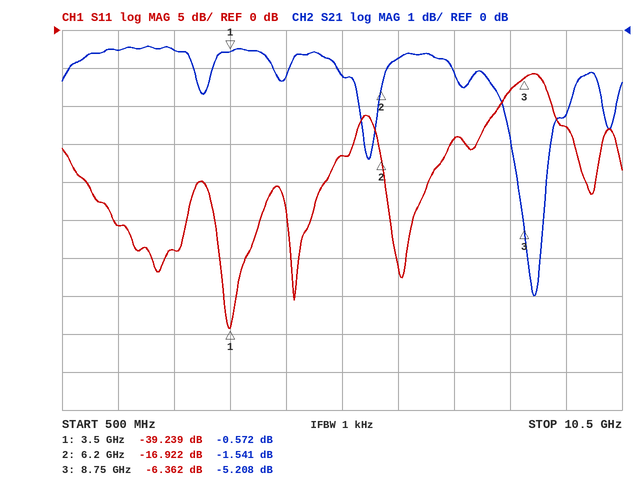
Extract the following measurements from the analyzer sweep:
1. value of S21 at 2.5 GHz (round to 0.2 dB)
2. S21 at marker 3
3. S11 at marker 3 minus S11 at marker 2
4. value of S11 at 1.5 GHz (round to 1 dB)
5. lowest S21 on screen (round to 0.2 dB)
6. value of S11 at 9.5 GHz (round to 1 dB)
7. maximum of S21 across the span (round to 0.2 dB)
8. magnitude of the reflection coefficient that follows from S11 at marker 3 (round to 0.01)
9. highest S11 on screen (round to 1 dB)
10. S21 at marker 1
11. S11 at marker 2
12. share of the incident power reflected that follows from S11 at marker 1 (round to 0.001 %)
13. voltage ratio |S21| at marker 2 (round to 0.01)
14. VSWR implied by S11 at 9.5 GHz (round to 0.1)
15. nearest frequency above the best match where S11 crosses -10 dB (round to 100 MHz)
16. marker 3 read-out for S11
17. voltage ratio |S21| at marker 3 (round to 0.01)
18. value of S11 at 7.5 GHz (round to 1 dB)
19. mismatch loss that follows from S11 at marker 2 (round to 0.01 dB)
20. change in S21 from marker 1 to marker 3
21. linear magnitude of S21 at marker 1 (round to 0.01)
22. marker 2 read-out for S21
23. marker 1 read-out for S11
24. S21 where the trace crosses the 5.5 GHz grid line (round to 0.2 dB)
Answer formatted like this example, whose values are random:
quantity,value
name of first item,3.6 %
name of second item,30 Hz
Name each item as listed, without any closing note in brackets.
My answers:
quantity,value
value of S21 at 2.5 GHz,-0.6 dB
S21 at marker 3,-5.208 dB
S11 at marker 3 minus S11 at marker 2,10.560 dB
value of S11 at 1.5 GHz,-26 dB
lowest S21 on screen,-7.0 dB
value of S11 at 9.5 GHz,-13 dB
maximum of S21 across the span,-0.4 dB
magnitude of the reflection coefficient that follows from S11 at marker 3,0.48
highest S11 on screen,-6 dB
S21 at marker 1,-0.572 dB
S11 at marker 2,-16.922 dB
share of the incident power reflected that follows from S11 at marker 1,0.012 %
voltage ratio |S21| at marker 2,0.84
VSWR implied by S11 at 9.5 GHz,1.6
nearest frequency above the best match where S11 crosses -10 dB,8.3 GHz
marker 3 read-out for S11,-6.362 dB
voltage ratio |S21| at marker 3,0.55
value of S11 at 7.5 GHz,-14 dB
mismatch loss that follows from S11 at marker 2,0.09 dB
change in S21 from marker 1 to marker 3,-4.636 dB
linear magnitude of S21 at marker 1,0.94
marker 2 read-out for S21,-1.541 dB
marker 1 read-out for S11,-39.239 dB
S21 where the trace crosses the 5.5 GHz grid line,-1.2 dB
